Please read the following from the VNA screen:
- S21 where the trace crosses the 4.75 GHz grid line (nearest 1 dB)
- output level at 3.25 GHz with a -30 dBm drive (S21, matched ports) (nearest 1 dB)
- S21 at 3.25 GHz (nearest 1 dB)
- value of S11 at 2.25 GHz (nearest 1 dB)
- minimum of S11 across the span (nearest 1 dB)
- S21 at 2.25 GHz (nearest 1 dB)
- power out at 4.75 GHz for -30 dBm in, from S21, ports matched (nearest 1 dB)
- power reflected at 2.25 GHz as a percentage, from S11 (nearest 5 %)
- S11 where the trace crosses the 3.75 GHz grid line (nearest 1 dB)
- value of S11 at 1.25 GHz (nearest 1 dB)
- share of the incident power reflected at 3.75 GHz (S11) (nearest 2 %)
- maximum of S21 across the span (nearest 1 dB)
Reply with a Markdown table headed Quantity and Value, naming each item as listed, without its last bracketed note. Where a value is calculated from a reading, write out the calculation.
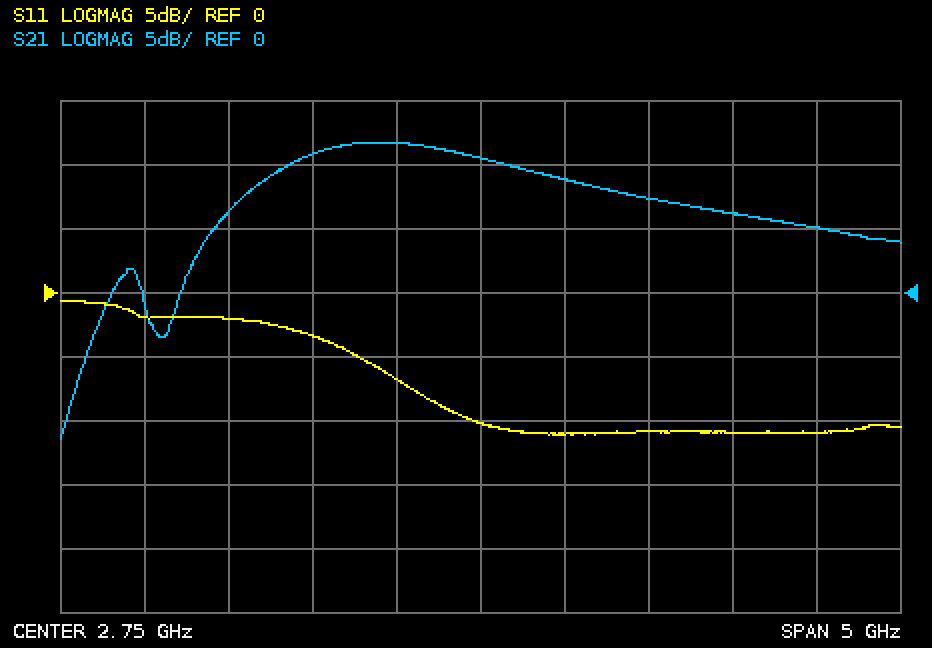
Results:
| Quantity | Value |
|---|---|
| S21 where the trace crosses the 4.75 GHz grid line | 5 dB |
| output level at 3.25 GHz with a -30 dBm drive (S21, matched ports) | -30 dBm + (9 dB) = -21 dBm |
| S21 at 3.25 GHz | 9 dB |
| value of S11 at 2.25 GHz | -7 dB |
| minimum of S11 across the span | -11 dB |
| S21 at 2.25 GHz | 12 dB |
| power out at 4.75 GHz for -30 dBm in, from S21, ports matched | -30 dBm + (5 dB) = -25 dBm |
| power reflected at 2.25 GHz as a percentage, from S11 | 10^(-7/10) ≈ 20 % |
| S11 where the trace crosses the 3.75 GHz grid line | -11 dB |
| value of S11 at 1.25 GHz | -2 dB |
| share of the incident power reflected at 3.75 GHz (S11) | 10^(-11/10) ≈ 8 % |
| maximum of S21 across the span | 12 dB |
